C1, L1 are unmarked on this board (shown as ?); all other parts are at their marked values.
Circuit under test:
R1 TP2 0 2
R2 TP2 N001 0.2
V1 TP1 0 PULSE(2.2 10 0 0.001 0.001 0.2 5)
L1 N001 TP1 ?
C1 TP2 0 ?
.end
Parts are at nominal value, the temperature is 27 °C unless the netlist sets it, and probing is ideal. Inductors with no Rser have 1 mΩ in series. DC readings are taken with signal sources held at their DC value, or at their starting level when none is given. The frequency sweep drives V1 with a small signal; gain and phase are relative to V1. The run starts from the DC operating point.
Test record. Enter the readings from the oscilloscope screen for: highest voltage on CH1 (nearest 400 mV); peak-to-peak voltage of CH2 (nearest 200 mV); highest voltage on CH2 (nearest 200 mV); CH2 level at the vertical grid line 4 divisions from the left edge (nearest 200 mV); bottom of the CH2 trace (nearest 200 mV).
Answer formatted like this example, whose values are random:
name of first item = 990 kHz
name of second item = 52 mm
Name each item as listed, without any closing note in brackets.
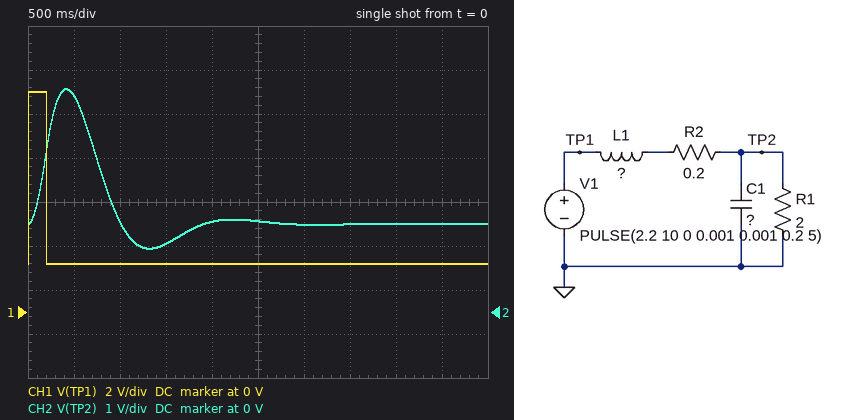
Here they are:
highest voltage on CH1 = 10.0 V
peak-to-peak voltage of CH2 = 3.6 V
highest voltage on CH2 = 5.0 V
CH2 level at the vertical grid line 4 divisions from the left edge = 2.0 V
bottom of the CH2 trace = 1.4 V
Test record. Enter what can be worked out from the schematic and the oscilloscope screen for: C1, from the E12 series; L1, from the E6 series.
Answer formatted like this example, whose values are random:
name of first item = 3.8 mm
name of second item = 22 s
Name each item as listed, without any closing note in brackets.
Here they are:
C1, from the E12 series = 150 mF
L1, from the E6 series = 470 mH
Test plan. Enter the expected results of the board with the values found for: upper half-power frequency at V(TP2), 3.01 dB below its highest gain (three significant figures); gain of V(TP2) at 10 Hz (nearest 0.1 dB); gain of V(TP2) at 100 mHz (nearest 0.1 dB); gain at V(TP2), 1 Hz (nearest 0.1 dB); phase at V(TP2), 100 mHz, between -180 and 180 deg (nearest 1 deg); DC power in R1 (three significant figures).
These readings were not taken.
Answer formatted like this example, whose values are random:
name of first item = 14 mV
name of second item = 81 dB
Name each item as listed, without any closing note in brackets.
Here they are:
upper half-power frequency at V(TP2), 3.01 dB below its highest gain = 740 mHz
gain of V(TP2) at 10 Hz = -48.9 dB
gain of V(TP2) at 100 mHz = -0.7 dB
gain at V(TP2), 1 Hz = -7.5 dB
phase at V(TP2), 100 mHz, between -180 and 180 deg = -9 deg
DC power in R1 = 2.00 W
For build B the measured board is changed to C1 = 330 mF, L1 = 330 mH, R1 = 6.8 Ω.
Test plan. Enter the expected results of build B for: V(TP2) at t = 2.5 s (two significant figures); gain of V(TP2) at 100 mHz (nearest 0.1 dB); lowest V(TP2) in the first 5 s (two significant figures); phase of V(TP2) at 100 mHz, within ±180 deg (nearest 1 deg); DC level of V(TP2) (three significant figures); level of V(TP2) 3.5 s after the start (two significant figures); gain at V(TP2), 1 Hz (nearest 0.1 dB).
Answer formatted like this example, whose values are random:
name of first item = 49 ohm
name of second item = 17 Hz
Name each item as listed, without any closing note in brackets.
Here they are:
V(TP2) at t = 2.5 s = 3.2 V
gain of V(TP2) at 100 mHz = 0.1 dB
lowest V(TP2) in the first 5 s = 46 mV
phase of V(TP2) at 100 mHz, within ±180 deg = -4 deg
DC level of V(TP2) = 2.14 V
level of V(TP2) 3.5 s after the start = 1.5 V
gain at V(TP2), 1 Hz = -10.5 dB
